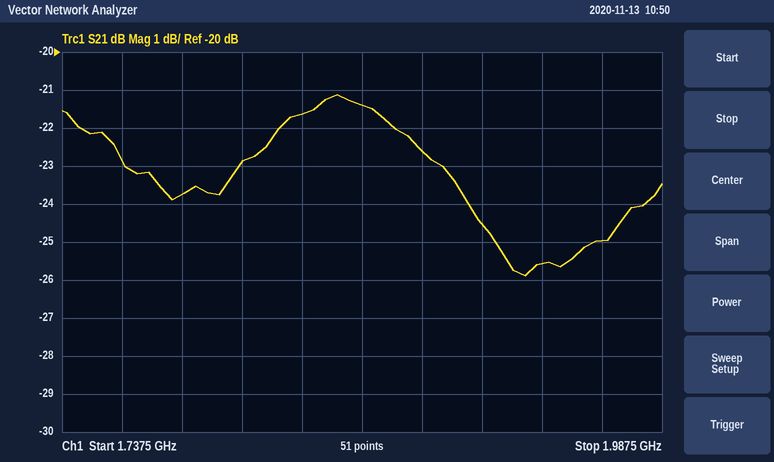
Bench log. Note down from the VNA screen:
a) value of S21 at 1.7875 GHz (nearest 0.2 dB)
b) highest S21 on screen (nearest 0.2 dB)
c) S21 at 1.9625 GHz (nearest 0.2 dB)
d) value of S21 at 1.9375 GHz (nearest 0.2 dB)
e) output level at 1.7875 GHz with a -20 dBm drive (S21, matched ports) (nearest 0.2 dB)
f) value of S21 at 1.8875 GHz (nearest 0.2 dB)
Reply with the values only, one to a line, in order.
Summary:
-23.8 dB
-21.2 dB
-25.0 dB
-25.6 dB
-43.8 dBm
-22.6 dB
